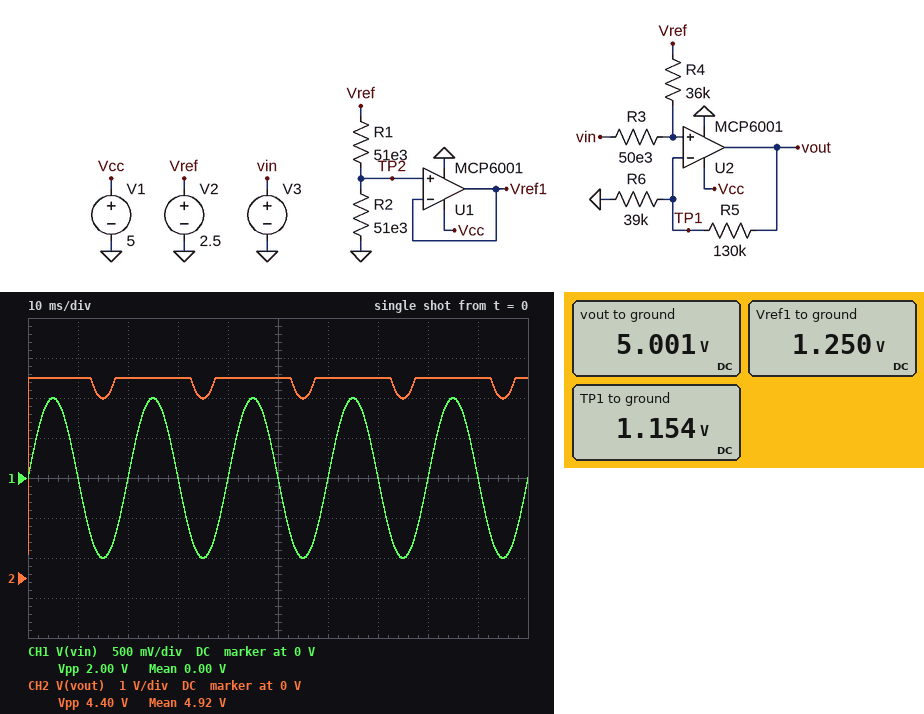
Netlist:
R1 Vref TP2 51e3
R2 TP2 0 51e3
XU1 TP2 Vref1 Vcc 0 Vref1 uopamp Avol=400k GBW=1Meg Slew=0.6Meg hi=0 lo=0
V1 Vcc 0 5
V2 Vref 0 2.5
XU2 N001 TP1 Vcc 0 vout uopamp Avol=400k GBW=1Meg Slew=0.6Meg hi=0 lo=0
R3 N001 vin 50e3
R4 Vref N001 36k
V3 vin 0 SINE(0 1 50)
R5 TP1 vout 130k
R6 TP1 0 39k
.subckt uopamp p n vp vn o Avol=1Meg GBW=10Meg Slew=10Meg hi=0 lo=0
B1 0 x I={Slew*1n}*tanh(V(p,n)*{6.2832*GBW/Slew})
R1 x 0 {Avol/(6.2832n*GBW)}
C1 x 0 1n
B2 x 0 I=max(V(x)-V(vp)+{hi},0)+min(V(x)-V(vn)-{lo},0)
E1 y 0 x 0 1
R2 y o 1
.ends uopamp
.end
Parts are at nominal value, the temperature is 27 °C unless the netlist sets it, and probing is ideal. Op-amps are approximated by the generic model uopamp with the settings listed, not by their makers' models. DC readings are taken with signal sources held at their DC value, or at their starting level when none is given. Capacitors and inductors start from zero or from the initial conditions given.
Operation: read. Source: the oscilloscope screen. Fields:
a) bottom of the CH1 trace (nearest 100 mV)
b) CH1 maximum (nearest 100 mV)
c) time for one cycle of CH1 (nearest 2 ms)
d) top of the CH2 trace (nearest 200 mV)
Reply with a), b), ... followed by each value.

a) -1.0 V
b) 1.0 V
c) 20 ms
d) 5.0 V
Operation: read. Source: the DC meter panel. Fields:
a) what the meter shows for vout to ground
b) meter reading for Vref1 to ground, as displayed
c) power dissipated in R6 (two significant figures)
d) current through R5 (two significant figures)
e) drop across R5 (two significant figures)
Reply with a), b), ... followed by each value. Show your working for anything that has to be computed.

a) 5.001 V
b) 1.250 V
c) (1.154 V)^2 / 39 kΩ = 34 µW
d) (5.001 V - 1.154 V) / 130 kΩ = 30 µA
e) 5.001 V - 1.154 V = 3.8 V
